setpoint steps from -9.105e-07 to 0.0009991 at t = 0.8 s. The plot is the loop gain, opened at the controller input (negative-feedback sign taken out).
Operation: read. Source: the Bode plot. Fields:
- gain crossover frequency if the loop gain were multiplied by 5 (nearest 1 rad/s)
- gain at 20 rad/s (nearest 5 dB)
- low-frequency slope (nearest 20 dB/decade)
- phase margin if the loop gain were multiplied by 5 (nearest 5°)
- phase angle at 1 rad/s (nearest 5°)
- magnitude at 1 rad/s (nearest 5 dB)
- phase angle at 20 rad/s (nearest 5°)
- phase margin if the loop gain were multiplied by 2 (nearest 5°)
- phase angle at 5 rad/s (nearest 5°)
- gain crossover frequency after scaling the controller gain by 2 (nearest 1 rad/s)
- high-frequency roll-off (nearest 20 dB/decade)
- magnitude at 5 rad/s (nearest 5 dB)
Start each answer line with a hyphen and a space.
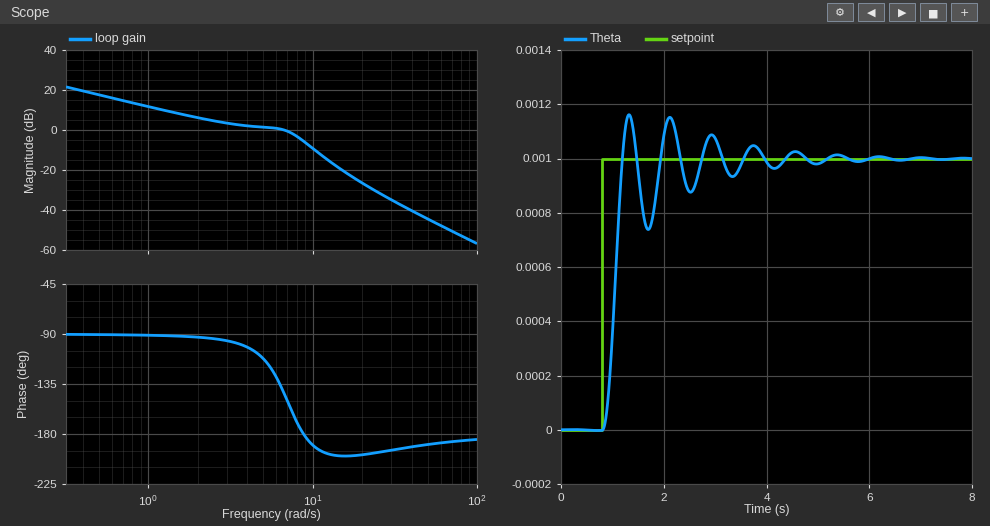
- 12 rad/s
- -25 dB
- -20 dB/decade
- -15°
- -90°
- 10 dB
- -200°
- 0°
- -110°
- 9 rad/s
- -40 dB/decade
- 0 dB
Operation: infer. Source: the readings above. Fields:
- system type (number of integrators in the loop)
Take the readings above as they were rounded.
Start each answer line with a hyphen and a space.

- 1
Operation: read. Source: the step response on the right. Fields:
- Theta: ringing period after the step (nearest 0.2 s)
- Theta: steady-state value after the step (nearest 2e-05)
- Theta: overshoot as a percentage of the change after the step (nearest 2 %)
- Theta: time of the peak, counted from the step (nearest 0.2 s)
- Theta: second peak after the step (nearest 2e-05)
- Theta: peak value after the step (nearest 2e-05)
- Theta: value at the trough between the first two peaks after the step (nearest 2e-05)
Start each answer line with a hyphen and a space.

- 0.8 s
- 0.00100
- 16 %
- 0.6 s
- 0.00116
- 0.00116
- 0.00074
